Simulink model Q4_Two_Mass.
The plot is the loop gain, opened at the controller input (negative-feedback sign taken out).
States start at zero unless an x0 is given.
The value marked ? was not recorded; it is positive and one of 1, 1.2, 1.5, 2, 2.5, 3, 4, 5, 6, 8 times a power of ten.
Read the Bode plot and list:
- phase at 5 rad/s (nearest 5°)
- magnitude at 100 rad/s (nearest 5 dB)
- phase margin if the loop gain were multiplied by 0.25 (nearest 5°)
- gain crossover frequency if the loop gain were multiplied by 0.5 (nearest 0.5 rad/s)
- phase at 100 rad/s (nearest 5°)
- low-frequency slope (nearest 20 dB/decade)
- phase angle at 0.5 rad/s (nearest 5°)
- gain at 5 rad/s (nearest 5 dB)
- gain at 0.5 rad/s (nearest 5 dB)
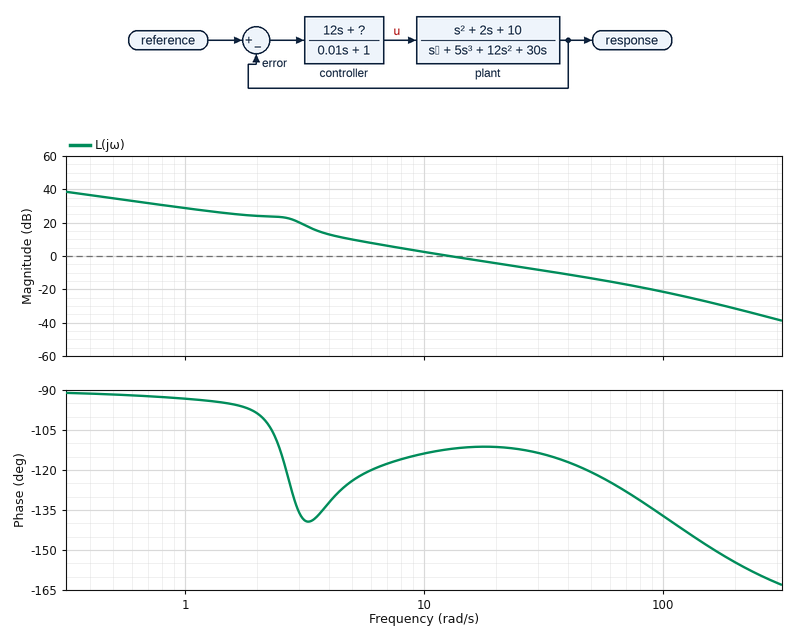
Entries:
-125°
-20 dB
50°
7.0 rad/s
-135°
-20 dB/decade
-90°
10 dB
35 dB
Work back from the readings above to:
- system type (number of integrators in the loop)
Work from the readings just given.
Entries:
1
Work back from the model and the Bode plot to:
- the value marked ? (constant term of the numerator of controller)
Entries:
80
